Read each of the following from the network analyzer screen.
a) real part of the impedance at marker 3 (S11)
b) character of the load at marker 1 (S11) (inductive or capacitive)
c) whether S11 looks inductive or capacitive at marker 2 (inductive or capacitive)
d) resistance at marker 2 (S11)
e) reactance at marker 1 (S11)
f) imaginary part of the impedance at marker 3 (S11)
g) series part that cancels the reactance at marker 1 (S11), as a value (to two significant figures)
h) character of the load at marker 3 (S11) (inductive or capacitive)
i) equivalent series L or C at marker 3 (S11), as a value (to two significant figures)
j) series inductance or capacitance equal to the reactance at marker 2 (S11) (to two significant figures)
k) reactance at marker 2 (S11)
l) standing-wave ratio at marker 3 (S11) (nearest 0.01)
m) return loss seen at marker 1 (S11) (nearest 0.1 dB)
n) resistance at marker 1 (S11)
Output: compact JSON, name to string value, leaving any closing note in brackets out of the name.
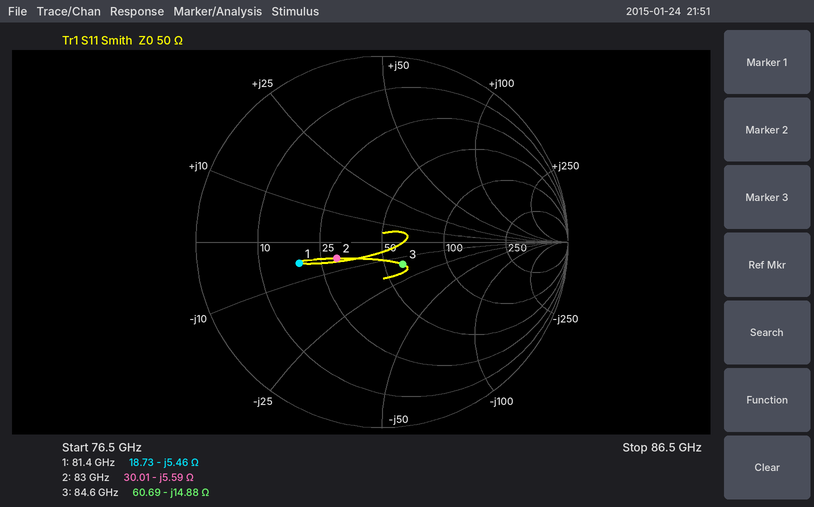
{"real part of the impedance at marker 3": "60.69 Ω", "character of the load at marker 1 (S11)": "capacitive", "whether S11 looks inductive or capacitive at marker 2": "capacitive", "resistance at marker 2": "30.01 Ω", "reactance at marker 1": "-5.46 Ω", "imaginary part of the impedance at marker 3": "-14.88 Ω", "series part that cancels the reactance at marker 1 (S11), as a value": "11 pH", "character of the load at marker 3 (S11)": "capacitive", "equivalent series L or C at marker 3 (S11), as a value": "130 fF", "series inductance or capacitance equal to the reactance at marker 2 (S11)": "340 fF", "reactance at marker 2": "-5.59 Ω", "standing-wave ratio at marker 3 (S11)": "1.39", "return loss seen at marker 1 (S11)": "6.7 dB", "resistance at marker 1": "18.73 Ω"}
